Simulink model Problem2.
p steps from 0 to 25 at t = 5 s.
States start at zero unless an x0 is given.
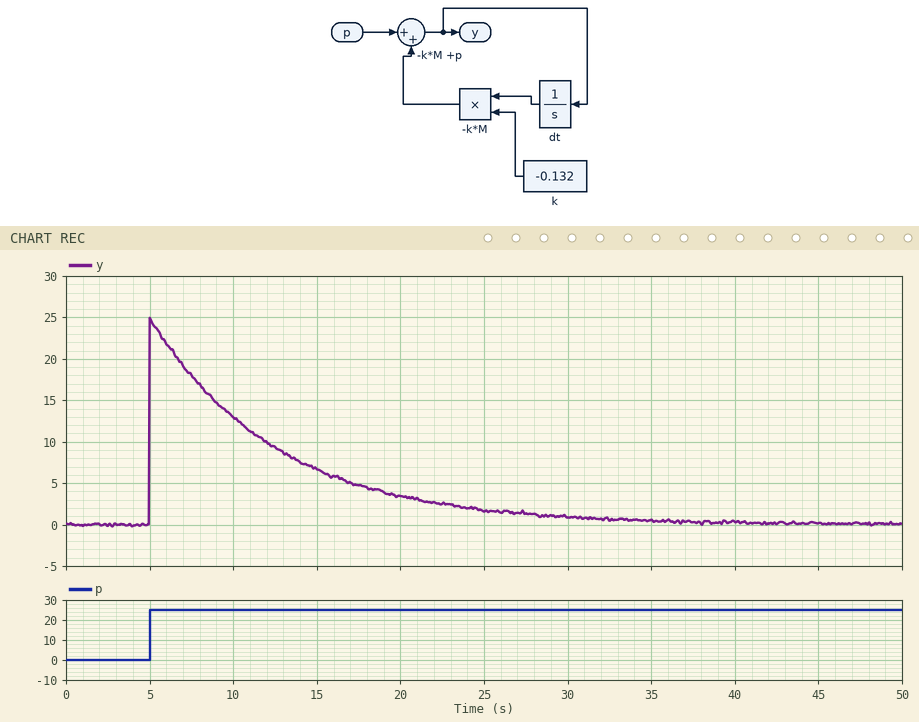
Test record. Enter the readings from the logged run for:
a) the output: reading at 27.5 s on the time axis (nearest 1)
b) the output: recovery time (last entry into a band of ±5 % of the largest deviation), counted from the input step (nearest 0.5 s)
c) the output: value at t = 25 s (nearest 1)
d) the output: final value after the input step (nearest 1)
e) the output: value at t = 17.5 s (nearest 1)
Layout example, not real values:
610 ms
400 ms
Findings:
1
22.5 s
2
0
5
